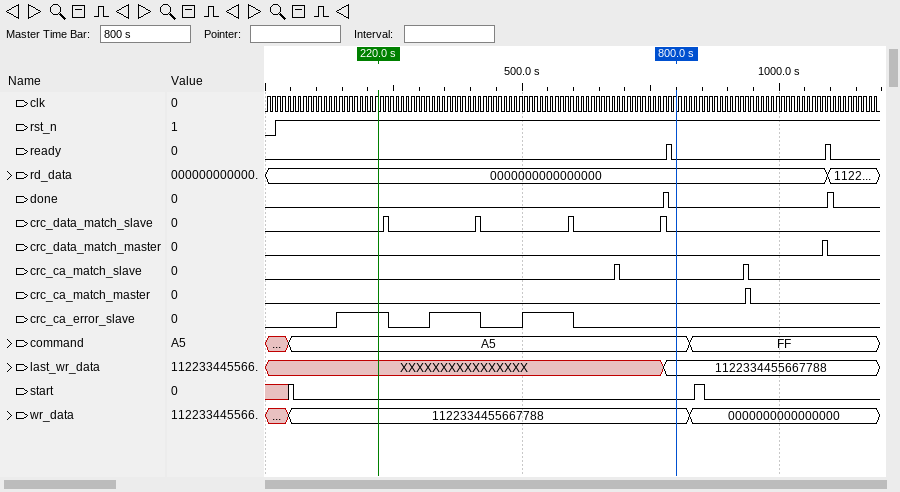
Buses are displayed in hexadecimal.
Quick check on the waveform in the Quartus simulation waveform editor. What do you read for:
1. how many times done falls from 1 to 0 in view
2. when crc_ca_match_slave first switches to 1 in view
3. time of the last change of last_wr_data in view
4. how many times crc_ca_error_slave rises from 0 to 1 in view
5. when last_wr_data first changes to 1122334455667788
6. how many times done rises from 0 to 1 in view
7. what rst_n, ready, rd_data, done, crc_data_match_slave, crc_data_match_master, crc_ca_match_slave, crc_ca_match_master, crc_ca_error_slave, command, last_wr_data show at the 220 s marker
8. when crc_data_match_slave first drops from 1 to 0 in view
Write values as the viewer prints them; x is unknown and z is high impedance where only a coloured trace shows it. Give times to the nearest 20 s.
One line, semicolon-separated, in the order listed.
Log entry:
2; 680 s; 780 s; 3; 780 s; 2; rst_n=1, ready=0, rd_data=0000000000000000, done=0, crc_data_match_slave=0, crc_data_match_master=0, crc_ca_match_slave=0, crc_ca_match_master=0, crc_ca_error_slave=1, command=A5, last_wr_data=XXXXXXXXXXXXXXXX; 240 s
